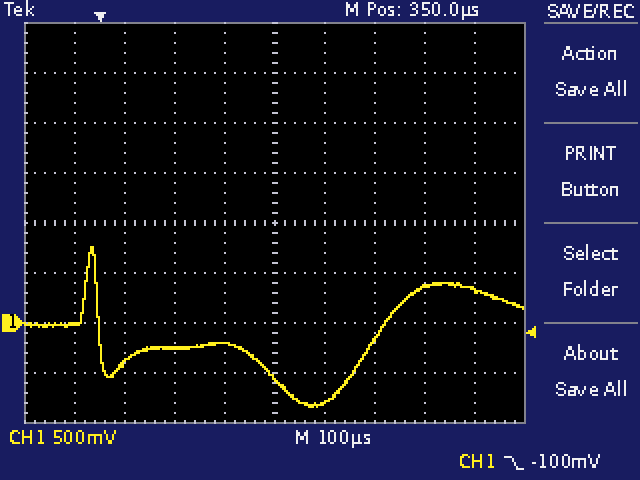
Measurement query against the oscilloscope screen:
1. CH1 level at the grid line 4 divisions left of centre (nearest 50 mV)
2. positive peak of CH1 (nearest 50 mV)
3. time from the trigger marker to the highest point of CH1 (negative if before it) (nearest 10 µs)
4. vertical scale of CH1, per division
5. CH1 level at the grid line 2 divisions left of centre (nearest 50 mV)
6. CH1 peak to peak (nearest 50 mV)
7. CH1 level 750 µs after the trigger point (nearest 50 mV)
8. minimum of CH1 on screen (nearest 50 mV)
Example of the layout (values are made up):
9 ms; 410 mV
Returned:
0 mV; 750 mV; -10 µs; 500 mV; -250 mV; 1.60 V; 350 mV; -850 mV
